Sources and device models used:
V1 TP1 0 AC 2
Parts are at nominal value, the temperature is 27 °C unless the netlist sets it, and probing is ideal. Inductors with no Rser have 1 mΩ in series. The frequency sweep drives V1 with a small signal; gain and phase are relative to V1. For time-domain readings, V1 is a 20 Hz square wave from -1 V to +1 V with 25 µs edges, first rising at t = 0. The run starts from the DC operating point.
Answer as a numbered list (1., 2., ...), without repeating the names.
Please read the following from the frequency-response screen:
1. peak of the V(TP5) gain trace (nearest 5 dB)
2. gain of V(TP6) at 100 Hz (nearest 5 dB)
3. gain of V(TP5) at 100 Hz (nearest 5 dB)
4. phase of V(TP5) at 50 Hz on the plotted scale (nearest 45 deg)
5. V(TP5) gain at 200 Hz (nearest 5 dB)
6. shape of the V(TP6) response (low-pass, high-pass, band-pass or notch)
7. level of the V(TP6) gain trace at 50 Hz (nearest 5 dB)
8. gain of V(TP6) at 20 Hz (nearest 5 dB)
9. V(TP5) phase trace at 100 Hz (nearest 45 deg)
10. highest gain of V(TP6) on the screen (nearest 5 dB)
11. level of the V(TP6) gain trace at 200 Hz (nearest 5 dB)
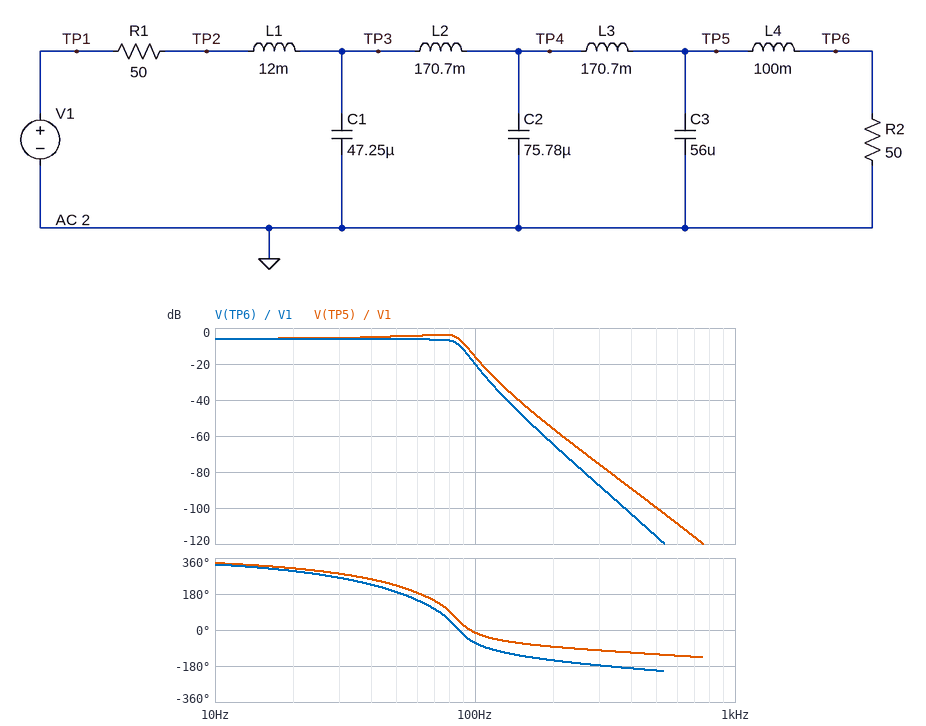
1. -5 dB
2. -20 dB
3. -15 dB
4. 225 deg
5. -55 dB
6. low-pass
7. -5 dB
8. -5 dB
9. 0 deg
10. -5 dB
11. -65 dB
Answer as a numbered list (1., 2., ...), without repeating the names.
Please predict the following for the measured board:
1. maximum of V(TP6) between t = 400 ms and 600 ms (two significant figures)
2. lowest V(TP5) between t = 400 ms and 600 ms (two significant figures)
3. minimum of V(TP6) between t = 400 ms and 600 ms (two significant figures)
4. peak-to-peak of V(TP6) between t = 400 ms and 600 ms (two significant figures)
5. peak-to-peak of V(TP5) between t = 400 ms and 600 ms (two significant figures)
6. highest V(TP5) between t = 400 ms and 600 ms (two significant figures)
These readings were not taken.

1. 650 mV
2. -740 mV
3. -650 mV
4. 1.3 V
5. 1.5 V
6. 740 mV
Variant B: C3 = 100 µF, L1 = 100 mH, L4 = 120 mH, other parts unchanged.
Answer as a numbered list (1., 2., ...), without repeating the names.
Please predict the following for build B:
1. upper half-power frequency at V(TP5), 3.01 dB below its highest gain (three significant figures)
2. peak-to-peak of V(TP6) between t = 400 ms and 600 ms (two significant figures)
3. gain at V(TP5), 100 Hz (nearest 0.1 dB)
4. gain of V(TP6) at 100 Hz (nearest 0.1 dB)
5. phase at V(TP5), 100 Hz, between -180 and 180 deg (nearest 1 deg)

1. 75.3 Hz
2. 1.3 V
3. -21.6 dB
4. -26.7 dB
5. -87 deg
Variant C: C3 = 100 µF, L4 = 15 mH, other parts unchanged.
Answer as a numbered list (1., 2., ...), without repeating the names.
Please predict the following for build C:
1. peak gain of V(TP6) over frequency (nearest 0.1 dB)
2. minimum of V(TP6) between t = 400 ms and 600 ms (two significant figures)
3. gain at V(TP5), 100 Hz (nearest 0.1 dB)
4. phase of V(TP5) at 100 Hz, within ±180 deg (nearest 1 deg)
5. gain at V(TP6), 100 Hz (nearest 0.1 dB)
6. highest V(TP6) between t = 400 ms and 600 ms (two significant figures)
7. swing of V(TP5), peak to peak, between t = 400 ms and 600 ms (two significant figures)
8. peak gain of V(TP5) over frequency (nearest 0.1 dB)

1. -6.0 dB
2. -600 mV
3. -26.3 dB
4. -22 deg
5. -26.5 dB
6. 600 mV
7. 1.2 V
8. -6.0 dB
